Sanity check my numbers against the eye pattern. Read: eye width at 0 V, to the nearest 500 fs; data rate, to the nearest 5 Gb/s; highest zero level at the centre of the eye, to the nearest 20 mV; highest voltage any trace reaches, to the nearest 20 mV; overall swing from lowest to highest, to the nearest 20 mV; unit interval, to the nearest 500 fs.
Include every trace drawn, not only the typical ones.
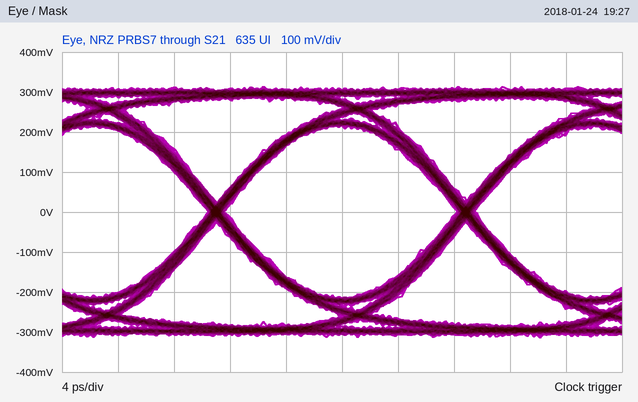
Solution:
16.5 ps
55 Gb/s
-220 mV
320 mV
620 mV
18.0 ps
